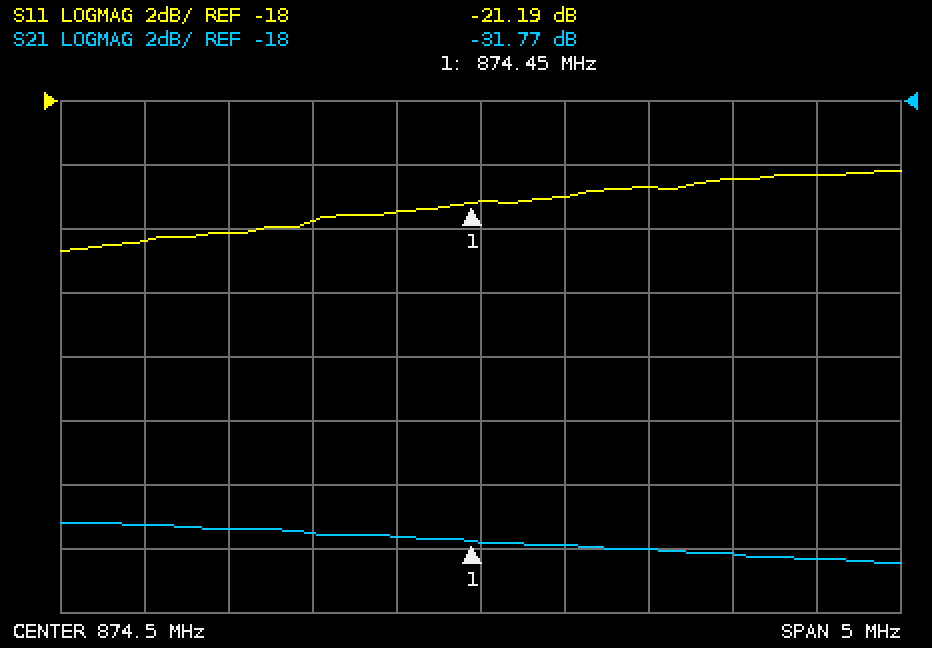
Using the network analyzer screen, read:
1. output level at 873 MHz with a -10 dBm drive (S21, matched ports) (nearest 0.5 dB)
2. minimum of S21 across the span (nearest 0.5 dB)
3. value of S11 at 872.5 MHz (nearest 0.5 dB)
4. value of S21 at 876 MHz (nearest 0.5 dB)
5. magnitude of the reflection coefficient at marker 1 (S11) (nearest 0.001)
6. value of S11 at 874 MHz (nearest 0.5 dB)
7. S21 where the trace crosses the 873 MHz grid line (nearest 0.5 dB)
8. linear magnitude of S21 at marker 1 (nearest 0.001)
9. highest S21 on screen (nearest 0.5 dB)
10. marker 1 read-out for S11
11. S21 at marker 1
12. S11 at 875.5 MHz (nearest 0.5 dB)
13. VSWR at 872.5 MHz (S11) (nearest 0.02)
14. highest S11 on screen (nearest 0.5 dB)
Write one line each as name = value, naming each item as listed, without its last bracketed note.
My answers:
output level at 873 MHz with a -10 dBm drive (S21, matched ports) = -41.5 dBm
minimum of S21 across the span = -32.5 dB
value of S11 at 872.5 MHz = -22.5 dB
value of S21 at 876 MHz = -32.0 dB
magnitude of the reflection coefficient at marker 1 (S11) = 0.087
value of S11 at 874 MHz = -21.5 dB
S21 where the trace crosses the 873 MHz grid line = -31.5 dB
linear magnitude of S21 at marker 1 = 0.026
highest S21 on screen = -31.0 dB
marker 1 read-out for S11 = -21.19 dB
S21 at marker 1 = -31.77 dB
S11 at 875.5 MHz = -20.5 dB
VSWR at 872.5 MHz (S11) = 1.16
highest S11 on screen = -20.0 dB
